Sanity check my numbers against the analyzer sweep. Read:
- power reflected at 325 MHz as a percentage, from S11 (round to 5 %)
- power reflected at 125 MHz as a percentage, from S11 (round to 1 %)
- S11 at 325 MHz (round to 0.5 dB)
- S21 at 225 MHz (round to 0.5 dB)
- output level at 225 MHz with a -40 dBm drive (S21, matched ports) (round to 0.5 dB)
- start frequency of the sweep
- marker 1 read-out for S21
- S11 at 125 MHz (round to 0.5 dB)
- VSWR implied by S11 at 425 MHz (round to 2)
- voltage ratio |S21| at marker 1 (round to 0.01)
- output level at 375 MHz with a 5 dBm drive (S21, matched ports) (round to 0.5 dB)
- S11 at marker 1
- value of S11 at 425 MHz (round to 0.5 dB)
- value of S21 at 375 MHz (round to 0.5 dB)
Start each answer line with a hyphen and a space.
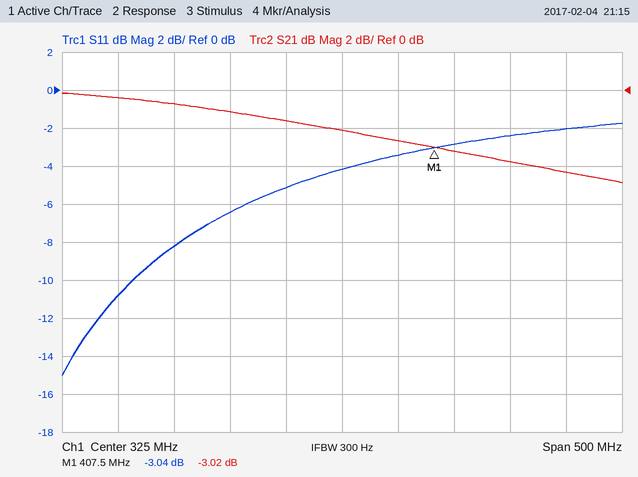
- 40 %
- 8 %
- -4.0 dB
- -1.0 dB
- -41.0 dBm
- 75 MHz
- -3.02 dB
- -11.0 dB
- 6
- 0.71
- 2.5 dBm
- -3.04 dB
- -3.0 dB
- -2.5 dB
